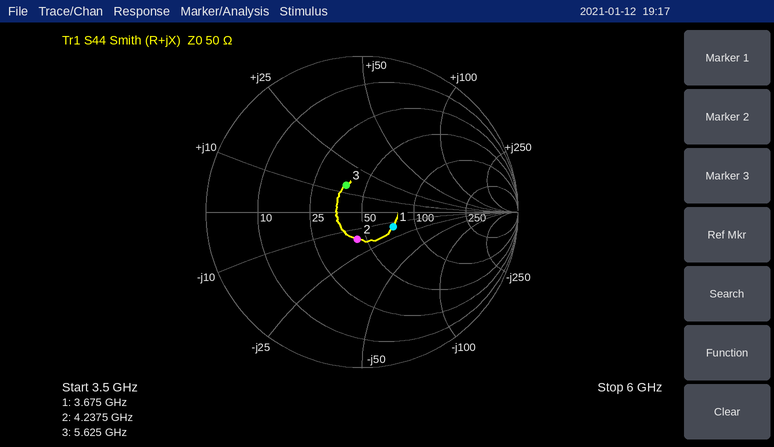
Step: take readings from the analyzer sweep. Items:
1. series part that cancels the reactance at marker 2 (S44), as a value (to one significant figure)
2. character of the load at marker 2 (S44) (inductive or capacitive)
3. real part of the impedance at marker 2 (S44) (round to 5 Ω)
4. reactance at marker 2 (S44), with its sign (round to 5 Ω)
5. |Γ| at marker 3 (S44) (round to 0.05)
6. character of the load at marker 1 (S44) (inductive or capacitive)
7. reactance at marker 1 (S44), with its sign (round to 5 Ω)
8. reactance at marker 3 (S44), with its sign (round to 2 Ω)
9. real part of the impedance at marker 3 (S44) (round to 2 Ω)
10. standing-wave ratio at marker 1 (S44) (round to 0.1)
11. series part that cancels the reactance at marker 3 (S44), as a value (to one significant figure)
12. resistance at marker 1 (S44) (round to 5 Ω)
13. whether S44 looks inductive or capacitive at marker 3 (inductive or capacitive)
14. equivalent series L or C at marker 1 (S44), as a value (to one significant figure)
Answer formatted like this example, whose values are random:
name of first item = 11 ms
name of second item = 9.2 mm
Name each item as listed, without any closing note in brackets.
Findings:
series part that cancels the reactance at marker 2 (S44), as a value = 600 pH
character of the load at marker 2 (S44) = capacitive
real part of the impedance at marker 2 (S44) = 45 Ω
reactance at marker 2 (S44), with its sign = -15 Ω
|Γ| at marker 3 (S44) = 0.20
character of the load at marker 1 (S44) = capacitive
reactance at marker 1 (S44), with its sign = -15 Ω
reactance at marker 3 (S44), with its sign = +14 Ω
real part of the impedance at marker 3 (S44) = 38 Ω
standing-wave ratio at marker 1 (S44) = 1.6
series part that cancels the reactance at marker 3 (S44), as a value = 2 pF
resistance at marker 1 (S44) = 75 Ω
whether S44 looks inductive or capacitive at marker 3 = inductive
equivalent series L or C at marker 1 (S44), as a value = 3 pF
